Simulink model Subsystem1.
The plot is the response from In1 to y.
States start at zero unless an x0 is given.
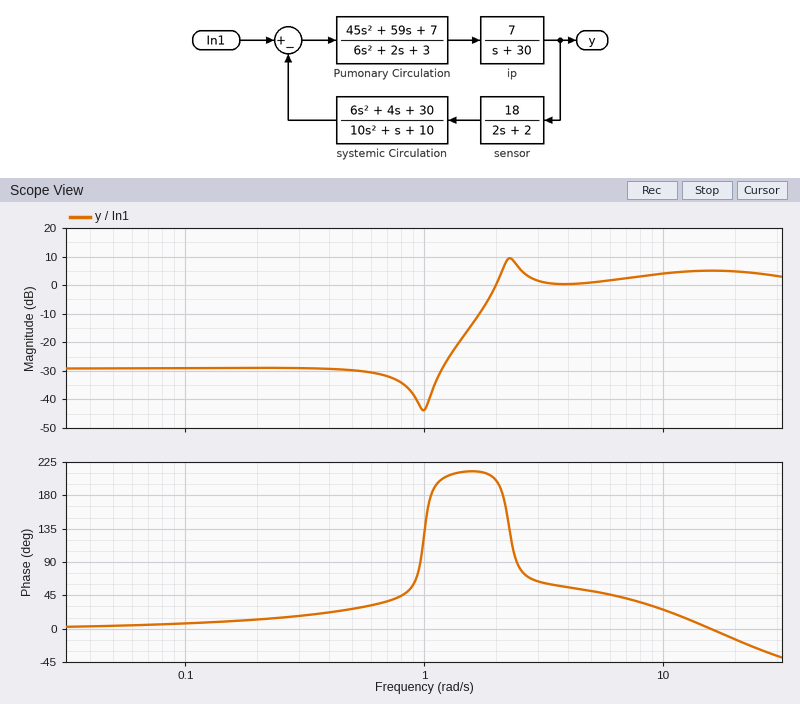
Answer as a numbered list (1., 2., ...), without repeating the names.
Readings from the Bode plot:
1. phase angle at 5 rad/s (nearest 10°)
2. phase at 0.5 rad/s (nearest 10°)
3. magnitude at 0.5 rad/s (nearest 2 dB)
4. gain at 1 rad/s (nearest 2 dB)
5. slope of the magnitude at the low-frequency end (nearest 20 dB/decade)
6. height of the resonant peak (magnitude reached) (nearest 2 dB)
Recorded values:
1. 50°
2. 30°
3. -30 dB
4. -44 dB
5. 0 dB/decade
6. 10 dB
